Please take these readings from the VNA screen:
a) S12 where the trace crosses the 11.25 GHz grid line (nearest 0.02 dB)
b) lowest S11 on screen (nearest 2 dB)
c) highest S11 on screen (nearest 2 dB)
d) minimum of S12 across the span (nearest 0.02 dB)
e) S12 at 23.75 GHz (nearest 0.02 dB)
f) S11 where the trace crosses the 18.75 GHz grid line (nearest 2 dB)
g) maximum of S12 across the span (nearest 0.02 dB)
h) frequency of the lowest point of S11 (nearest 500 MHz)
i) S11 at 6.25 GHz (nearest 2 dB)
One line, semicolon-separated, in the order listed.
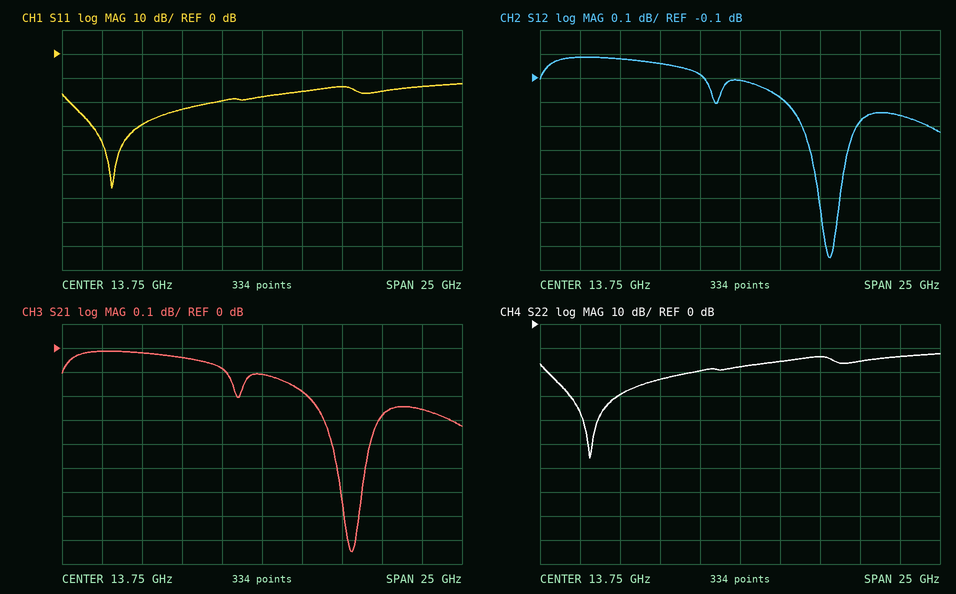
-0.08 dB; -56 dB; -12 dB; -0.84 dB; -0.26 dB; -14 dB; -0.02 dB; 4.5 GHz; -30 dB
